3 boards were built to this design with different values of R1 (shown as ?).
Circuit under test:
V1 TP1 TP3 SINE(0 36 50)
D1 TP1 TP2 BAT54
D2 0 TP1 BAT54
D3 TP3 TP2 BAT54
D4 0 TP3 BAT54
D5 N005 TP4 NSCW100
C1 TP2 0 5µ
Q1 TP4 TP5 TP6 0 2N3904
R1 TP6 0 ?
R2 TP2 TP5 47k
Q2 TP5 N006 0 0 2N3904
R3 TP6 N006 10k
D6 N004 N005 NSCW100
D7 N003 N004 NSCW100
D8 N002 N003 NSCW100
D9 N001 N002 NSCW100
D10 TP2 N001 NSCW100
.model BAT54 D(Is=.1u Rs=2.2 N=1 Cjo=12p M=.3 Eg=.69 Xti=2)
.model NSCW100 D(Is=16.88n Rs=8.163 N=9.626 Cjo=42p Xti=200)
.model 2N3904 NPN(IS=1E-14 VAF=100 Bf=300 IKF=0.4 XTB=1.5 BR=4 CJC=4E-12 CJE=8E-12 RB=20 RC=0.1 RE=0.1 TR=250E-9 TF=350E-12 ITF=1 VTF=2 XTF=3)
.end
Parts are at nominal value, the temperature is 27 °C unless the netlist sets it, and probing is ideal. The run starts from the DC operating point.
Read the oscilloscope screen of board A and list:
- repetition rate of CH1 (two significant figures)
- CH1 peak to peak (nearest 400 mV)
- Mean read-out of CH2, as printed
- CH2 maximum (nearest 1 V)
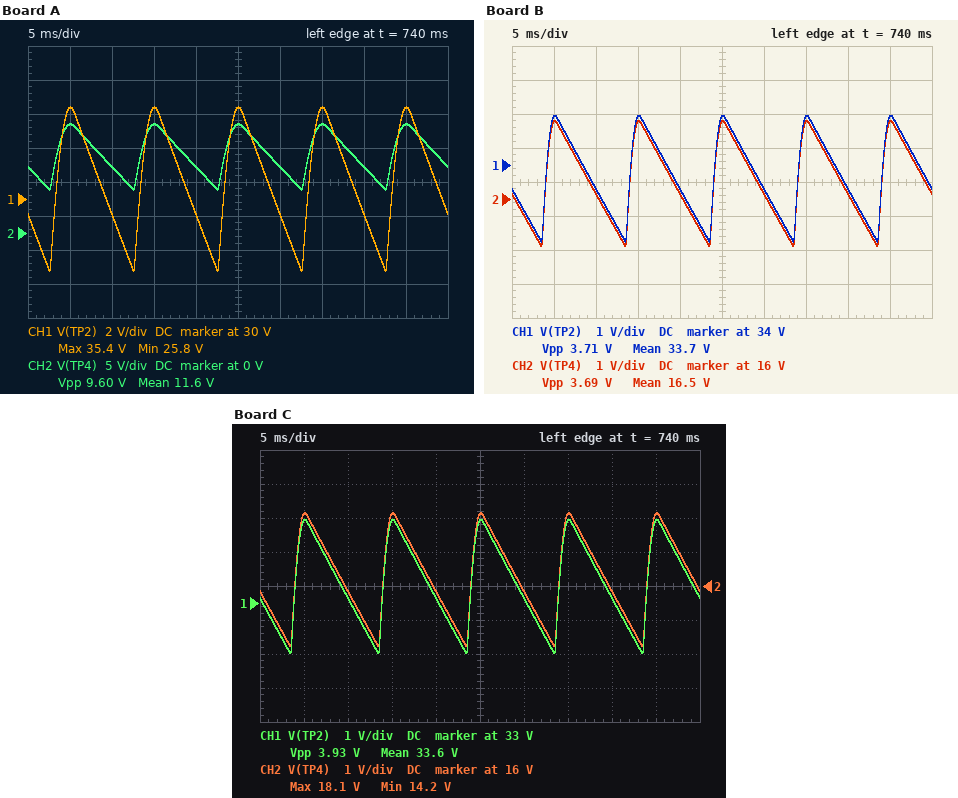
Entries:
100 Hz
9.6 V
11.6 V
16 V
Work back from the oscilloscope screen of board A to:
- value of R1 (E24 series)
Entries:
110 Ω
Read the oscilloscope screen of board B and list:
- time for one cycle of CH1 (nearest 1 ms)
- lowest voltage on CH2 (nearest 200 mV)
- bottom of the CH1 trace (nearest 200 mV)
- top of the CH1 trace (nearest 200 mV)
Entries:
10 ms
14.6 V
31.8 V
35.4 V
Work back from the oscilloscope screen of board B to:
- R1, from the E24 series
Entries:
430 Ω
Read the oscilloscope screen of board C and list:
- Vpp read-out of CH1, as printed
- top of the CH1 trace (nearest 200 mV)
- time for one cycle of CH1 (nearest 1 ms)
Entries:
3.93 V
35.4 V
10 ms
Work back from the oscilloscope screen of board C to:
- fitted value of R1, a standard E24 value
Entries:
390 Ω
